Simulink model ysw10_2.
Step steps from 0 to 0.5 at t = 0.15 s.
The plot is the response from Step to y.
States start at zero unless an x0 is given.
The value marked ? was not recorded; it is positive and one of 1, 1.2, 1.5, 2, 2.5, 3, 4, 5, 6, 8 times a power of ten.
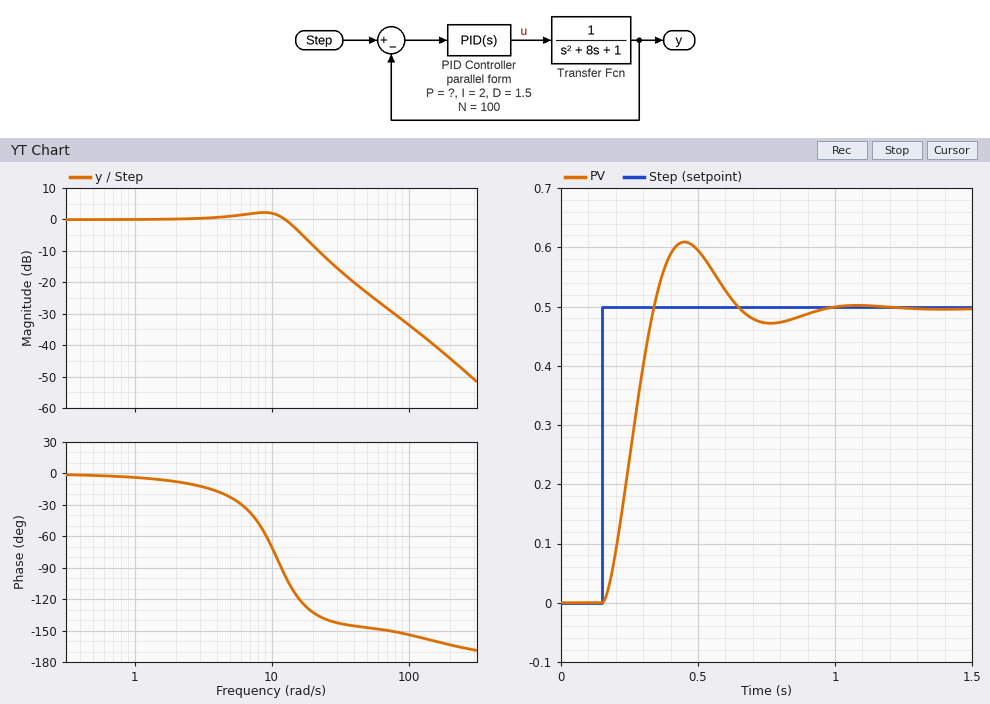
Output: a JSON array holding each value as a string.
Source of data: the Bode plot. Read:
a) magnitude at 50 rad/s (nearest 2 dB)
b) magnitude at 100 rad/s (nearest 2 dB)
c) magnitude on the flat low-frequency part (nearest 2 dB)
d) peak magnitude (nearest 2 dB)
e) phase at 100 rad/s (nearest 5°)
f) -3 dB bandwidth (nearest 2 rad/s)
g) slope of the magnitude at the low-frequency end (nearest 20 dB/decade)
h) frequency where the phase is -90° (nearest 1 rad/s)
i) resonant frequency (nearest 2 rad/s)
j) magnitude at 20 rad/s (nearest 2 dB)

["-24 dB", "-34 dB", "0 dB", "2 dB", "-155°", "16 rad/s", "0 dB/decade", "12 rad/s", "8 rad/s", "-8 dB"]
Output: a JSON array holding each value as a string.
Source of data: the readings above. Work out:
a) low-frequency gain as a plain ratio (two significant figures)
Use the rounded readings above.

["1.0"]
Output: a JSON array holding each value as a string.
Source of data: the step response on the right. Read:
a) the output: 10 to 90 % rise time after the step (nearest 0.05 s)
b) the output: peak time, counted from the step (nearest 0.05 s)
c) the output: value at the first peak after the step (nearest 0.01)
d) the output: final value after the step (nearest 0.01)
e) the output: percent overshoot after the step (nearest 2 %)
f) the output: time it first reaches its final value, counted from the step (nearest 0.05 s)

["0.15 s", "0.30 s", "0.61", "0.50", "22 %", "0.20 s"]
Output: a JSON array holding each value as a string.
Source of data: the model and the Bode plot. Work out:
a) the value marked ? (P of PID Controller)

["120"]
